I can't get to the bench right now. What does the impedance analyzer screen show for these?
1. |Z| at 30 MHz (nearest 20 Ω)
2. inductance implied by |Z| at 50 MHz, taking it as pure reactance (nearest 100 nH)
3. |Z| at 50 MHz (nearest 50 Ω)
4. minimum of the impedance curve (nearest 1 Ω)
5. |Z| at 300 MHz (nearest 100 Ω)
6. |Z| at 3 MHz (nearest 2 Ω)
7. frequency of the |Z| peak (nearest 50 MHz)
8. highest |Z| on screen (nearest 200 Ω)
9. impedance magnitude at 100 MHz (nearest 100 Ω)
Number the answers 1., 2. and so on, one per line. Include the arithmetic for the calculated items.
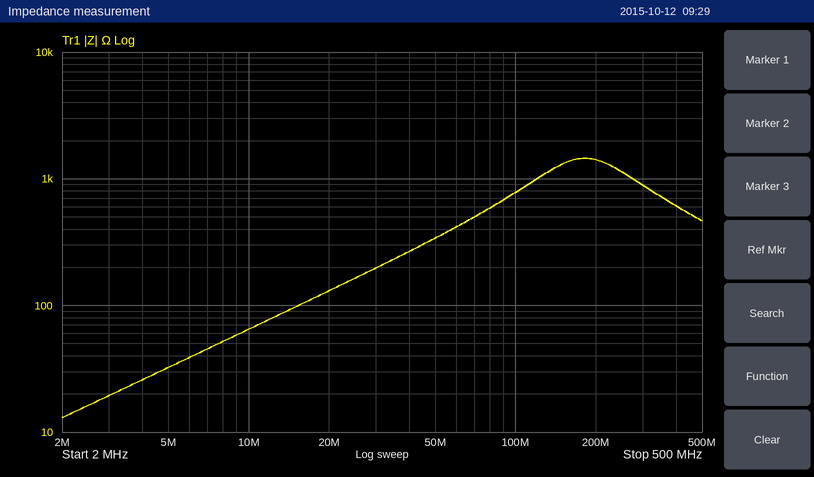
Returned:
1. 200 Ω
2. L = 350 Ω/(2π × 50 MHz) ≈ 1.1 µH
3. 350 Ω
4. 13 Ω
5. 900 Ω
6. 20 Ω
7. 200 MHz
8. 1.4 kΩ
9. 800 Ω
